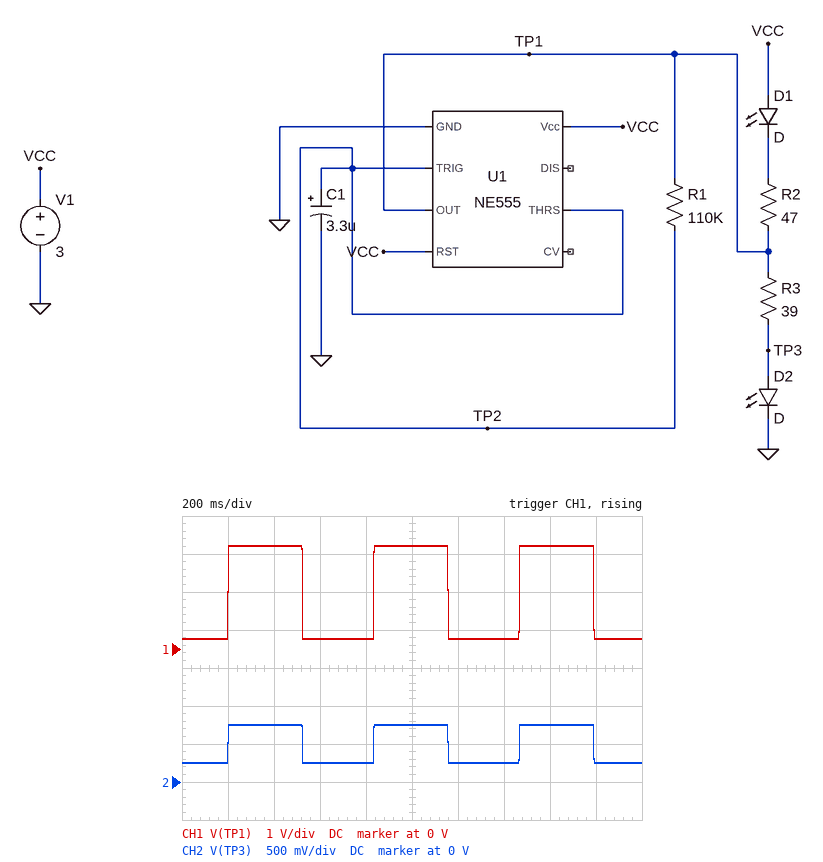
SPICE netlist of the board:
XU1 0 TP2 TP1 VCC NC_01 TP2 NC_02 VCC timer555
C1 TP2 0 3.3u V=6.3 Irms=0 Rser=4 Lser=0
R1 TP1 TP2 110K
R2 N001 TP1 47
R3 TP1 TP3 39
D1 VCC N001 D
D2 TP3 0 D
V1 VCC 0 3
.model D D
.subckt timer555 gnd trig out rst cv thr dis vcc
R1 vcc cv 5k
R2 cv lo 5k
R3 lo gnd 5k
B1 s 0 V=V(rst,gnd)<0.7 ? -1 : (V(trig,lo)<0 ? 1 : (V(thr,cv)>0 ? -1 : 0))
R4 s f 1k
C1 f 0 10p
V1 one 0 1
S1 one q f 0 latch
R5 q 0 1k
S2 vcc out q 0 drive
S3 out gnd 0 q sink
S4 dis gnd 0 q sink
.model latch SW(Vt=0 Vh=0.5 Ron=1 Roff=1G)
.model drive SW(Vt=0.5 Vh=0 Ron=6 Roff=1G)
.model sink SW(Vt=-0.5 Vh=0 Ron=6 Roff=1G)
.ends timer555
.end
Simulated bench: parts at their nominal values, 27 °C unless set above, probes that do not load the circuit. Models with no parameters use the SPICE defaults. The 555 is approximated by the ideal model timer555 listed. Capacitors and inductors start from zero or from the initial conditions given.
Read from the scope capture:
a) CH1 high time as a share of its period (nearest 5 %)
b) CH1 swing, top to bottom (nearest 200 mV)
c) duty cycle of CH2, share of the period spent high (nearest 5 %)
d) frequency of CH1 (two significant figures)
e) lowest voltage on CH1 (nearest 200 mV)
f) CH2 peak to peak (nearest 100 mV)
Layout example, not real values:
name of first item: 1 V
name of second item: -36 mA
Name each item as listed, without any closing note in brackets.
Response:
CH1 high time as a share of its period: 50 %
CH1 swing, top to bottom: 2.4 V
duty cycle of CH2, share of the period spent high: 50 %
frequency of CH1: 1.6 Hz
lowest voltage on CH1: 200 mV
CH2 peak to peak: 500 mV
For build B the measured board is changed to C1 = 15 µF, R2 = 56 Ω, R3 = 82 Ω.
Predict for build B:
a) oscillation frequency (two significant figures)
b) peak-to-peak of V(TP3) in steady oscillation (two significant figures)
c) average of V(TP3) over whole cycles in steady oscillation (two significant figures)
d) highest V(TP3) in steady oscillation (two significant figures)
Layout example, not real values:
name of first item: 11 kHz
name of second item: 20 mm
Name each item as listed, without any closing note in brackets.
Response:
oscillation frequency: 380 mHz
peak-to-peak of V(TP3) in steady oscillation: 520 mV
average of V(TP3) over whole cycles in steady oscillation: 470 mV
highest V(TP3) in steady oscillation: 740 mV
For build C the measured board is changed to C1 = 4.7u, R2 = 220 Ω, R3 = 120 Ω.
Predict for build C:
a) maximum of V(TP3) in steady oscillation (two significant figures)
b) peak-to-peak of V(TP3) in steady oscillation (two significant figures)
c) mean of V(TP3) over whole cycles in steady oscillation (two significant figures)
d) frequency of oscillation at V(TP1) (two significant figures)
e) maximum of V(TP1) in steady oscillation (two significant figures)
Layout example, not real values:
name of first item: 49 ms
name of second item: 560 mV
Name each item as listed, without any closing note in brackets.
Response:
maximum of V(TP3) in steady oscillation: 730 mV
peak-to-peak of V(TP3) in steady oscillation: 670 mV
mean of V(TP3) over whole cycles in steady oscillation: 400 mV
frequency of oscillation at V(TP1): 1.3 Hz
maximum of V(TP1) in steady oscillation: 2.9 V
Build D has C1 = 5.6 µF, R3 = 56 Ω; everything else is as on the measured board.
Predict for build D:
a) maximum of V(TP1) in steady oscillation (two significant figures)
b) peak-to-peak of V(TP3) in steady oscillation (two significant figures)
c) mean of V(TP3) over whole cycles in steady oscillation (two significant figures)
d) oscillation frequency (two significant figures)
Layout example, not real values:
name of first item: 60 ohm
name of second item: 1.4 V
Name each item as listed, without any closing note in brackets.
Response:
maximum of V(TP1) in steady oscillation: 2.8 V
peak-to-peak of V(TP3) in steady oscillation: 490 mV
mean of V(TP3) over whole cycles in steady oscillation: 500 mV
oscillation frequency: 970 mHz
